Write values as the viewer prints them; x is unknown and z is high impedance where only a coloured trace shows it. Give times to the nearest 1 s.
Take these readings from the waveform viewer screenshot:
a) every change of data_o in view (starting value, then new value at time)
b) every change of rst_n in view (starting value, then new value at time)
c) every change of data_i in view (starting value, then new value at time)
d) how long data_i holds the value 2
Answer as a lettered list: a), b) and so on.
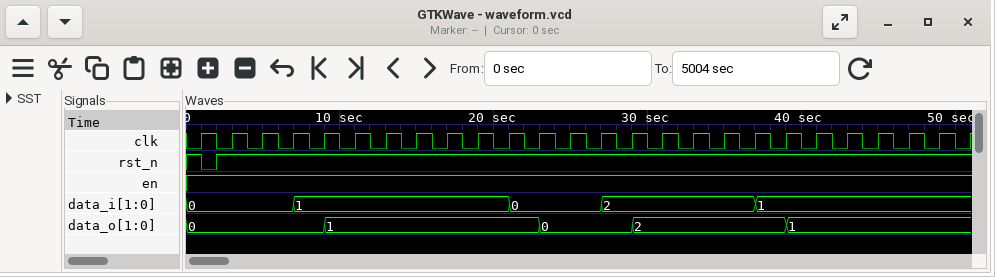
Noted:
a) 0, 1 at 9 s, 0 at 23 s, 2 at 29 s, 1 at 39 s
b) 1, 0 at 1 s, 1 at 2 s
c) 0, 1 at 7 s, 0 at 21 s, 2 at 27 s, 1 at 37 s
d) 10 s
